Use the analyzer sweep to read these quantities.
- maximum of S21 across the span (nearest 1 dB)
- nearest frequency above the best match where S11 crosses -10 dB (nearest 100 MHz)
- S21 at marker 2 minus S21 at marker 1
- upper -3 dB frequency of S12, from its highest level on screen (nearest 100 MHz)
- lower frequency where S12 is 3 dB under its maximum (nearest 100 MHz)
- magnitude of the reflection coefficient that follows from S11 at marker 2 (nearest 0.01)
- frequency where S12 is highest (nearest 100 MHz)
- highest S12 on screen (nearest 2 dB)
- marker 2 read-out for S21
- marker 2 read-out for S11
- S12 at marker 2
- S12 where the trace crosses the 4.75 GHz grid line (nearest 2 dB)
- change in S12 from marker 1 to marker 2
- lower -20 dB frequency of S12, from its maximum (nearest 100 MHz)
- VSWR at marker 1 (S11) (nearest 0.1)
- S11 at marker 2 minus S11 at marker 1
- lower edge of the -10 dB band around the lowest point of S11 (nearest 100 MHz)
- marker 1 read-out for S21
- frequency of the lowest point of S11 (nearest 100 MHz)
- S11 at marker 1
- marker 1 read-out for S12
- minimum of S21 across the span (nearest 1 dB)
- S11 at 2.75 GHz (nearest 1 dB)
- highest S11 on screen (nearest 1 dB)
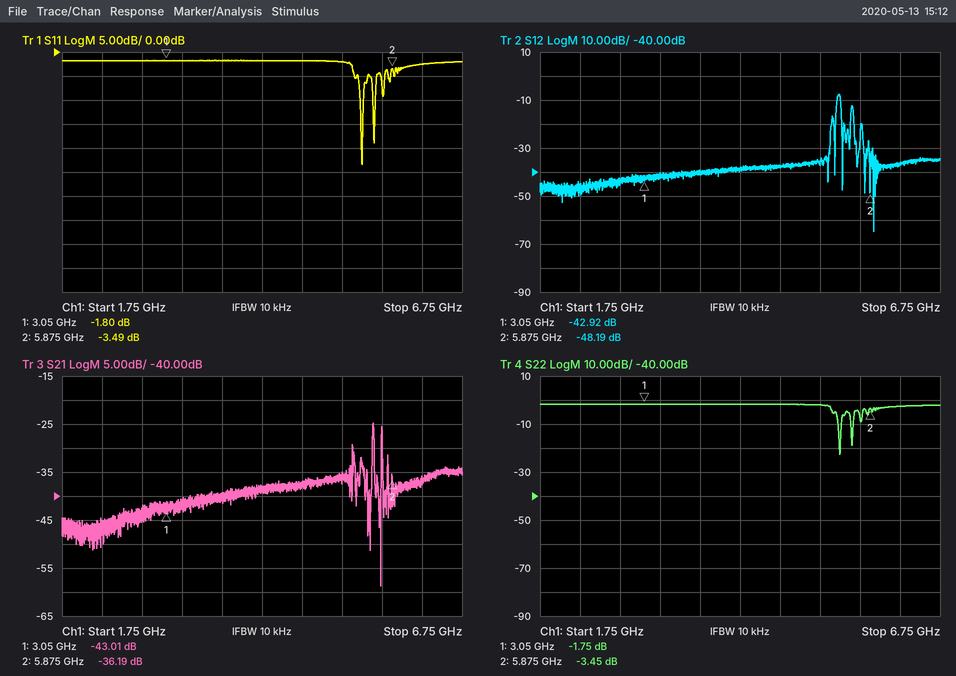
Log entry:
-25 dB
5.5 GHz
6.82 dB
5.5 GHz
5.5 GHz
0.67
5.5 GHz
-8 dB
-36.19 dB
-3.49 dB
-48.19 dB
-38 dB
-5.27 dB
5.4 GHz
9.7
-1.69 dB
5.5 GHz
-43.01 dB
5.5 GHz
-1.80 dB
-42.92 dB
-59 dB
-2 dB
-2 dB
